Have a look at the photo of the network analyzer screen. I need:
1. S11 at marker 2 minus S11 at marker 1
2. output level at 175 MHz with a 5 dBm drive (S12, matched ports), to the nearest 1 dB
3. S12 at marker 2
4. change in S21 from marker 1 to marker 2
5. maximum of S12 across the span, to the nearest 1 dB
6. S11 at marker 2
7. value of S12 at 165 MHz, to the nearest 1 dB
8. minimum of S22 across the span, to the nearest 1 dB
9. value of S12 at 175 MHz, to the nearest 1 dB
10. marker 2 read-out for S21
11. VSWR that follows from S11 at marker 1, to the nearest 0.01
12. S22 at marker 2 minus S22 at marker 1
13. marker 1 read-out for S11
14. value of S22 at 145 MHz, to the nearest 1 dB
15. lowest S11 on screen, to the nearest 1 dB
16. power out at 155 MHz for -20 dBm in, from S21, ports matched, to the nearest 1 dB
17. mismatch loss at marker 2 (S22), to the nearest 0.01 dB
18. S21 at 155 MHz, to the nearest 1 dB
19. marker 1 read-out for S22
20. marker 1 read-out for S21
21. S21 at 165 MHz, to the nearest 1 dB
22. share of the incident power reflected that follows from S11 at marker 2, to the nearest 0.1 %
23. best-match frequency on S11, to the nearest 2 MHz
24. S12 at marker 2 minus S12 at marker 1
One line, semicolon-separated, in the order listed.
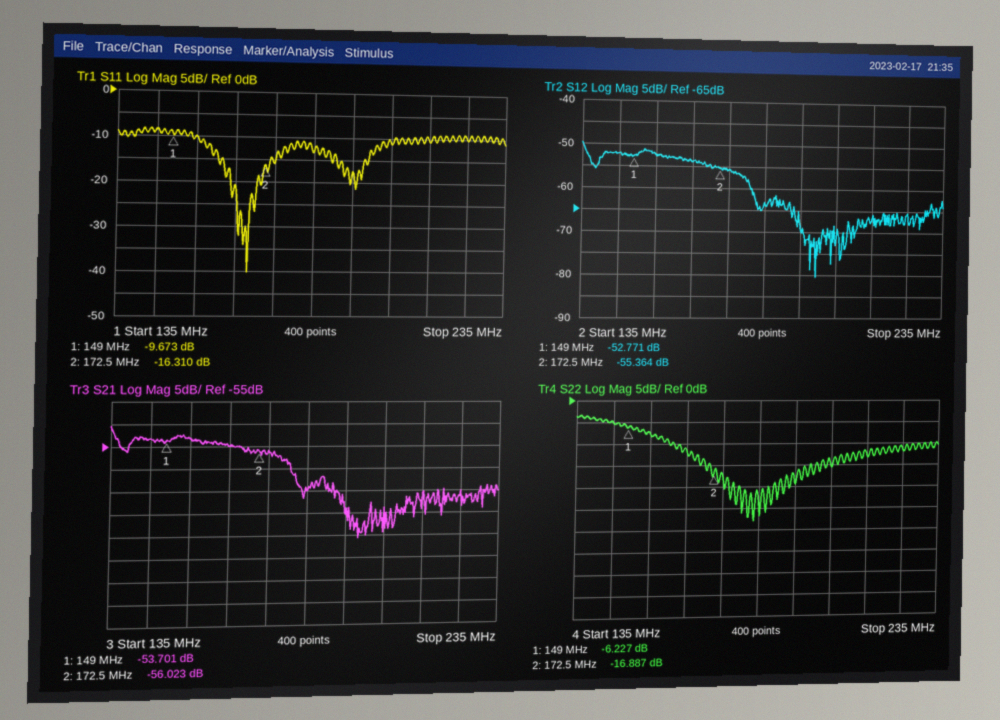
-6.637 dB; -51 dBm; -55.364 dB; -2.322 dB; -50 dB; -16.310 dB; -54 dB; -28 dB; -56 dB; -56.023 dB; 1.98; -10.660 dB; -9.673 dB; -5 dB; -40 dB; -73 dBm; 0.09 dB; -53 dB; -6.227 dB; -53.701 dB; -55 dB; 2.3 %; 168 MHz; -2.593 dB
